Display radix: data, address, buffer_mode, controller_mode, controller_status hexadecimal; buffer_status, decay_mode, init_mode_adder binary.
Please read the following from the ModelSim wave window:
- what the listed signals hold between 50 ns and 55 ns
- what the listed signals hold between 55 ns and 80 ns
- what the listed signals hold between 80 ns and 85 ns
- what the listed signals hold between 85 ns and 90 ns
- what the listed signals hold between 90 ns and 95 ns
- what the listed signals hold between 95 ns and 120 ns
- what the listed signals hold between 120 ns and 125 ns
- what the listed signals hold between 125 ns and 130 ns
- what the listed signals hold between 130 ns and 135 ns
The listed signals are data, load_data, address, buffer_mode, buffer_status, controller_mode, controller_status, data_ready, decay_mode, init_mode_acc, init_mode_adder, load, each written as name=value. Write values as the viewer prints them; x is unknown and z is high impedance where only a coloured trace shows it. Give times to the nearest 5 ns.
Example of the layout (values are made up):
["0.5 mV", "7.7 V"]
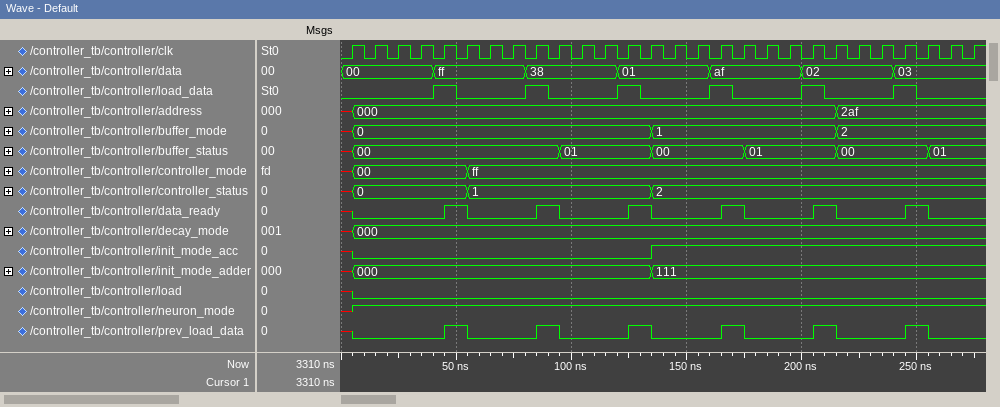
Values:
["data=ff, load_data=0, address=000, buffer_mode=0, buffer_status=00, controller_mode=00, controller_status=0, data_ready=1, decay_mode=000, init_mode_acc=0, init_mode_adder=000, load=0", "data=ff, load_data=0, address=000, buffer_mode=0, buffer_status=00, controller_mode=ff, controller_status=1, data_ready=0, decay_mode=000, init_mode_acc=0, init_mode_adder=000, load=0", "data=38, load_data=1, address=000, buffer_mode=0, buffer_status=00, controller_mode=ff, controller_status=1, data_ready=0, decay_mode=000, init_mode_acc=0, init_mode_adder=000, load=0", "data=38, load_data=1, address=000, buffer_mode=0, buffer_status=00, controller_mode=ff, controller_status=1, data_ready=1, decay_mode=000, init_mode_acc=0, init_mode_adder=000, load=0", "data=38, load_data=0, address=000, buffer_mode=0, buffer_status=00, controller_mode=ff, controller_status=1, data_ready=1, decay_mode=000, init_mode_acc=0, init_mode_adder=000, load=0", "data=38, load_data=0, address=000, buffer_mode=0, buffer_status=01, controller_mode=ff, controller_status=1, data_ready=0, decay_mode=000, init_mode_acc=0, init_mode_adder=000, load=0", "data=01, load_data=1, address=000, buffer_mode=0, buffer_status=01, controller_mode=ff, controller_status=1, data_ready=0, decay_mode=000, init_mode_acc=0, init_mode_adder=000, load=0", "data=01, load_data=1, address=000, buffer_mode=0, buffer_status=01, controller_mode=ff, controller_status=1, data_ready=1, decay_mode=000, init_mode_acc=0, init_mode_adder=000, load=0", "data=01, load_data=0, address=000, buffer_mode=0, buffer_status=01, controller_mode=ff, controller_status=1, data_ready=1, decay_mode=000, init_mode_acc=0, init_mode_adder=000, load=0"]
